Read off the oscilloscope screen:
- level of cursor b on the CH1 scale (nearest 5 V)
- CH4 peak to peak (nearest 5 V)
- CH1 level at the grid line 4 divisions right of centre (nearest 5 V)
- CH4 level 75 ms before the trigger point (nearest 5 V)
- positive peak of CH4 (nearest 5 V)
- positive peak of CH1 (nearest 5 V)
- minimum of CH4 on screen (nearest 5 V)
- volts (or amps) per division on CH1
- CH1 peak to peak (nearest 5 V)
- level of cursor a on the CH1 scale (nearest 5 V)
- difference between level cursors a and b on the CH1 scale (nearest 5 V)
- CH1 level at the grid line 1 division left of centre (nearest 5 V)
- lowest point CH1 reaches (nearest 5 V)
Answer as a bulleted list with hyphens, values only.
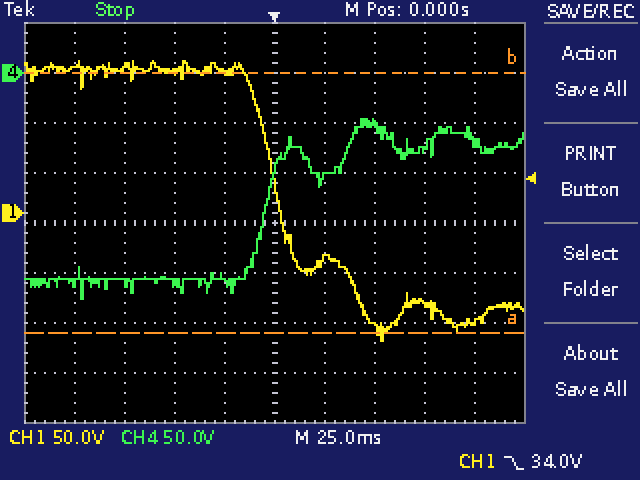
- 140 V
- 180 V
- -110 V
- -210 V
- -45 V
- 150 V
- -225 V
- 50 V
- 280 V
- -120 V
- 260 V
- 140 V
- -130 V
